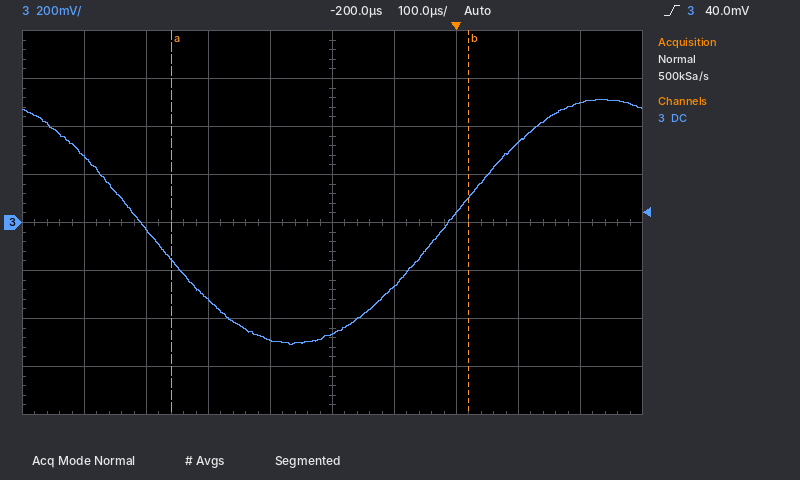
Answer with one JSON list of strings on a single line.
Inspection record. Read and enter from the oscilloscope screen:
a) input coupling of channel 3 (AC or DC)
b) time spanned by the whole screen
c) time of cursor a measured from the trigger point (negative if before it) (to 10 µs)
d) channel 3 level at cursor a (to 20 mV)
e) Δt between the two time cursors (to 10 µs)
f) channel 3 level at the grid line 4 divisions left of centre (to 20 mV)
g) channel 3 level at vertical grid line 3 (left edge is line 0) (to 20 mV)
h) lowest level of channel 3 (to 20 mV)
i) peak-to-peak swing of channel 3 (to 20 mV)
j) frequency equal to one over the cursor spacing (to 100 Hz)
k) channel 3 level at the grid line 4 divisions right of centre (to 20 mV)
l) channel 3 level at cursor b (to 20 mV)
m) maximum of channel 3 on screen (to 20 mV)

["DC", "1 ms", "-460 µs", "-160 mV", "480 µs", "280 mV", "-320 mV", "-500 mV", "1.02 V", "2.1 kHz", "500 mV", "100 mV", "520 mV"]
